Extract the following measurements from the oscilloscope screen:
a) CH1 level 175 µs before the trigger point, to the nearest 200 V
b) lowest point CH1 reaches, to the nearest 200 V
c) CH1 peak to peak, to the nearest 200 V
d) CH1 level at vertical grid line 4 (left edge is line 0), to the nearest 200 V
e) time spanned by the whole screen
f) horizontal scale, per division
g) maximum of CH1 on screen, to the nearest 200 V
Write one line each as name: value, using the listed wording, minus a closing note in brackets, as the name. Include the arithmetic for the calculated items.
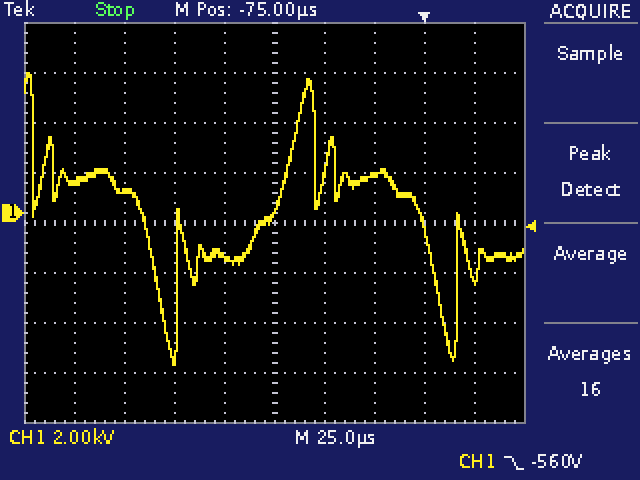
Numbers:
CH1 level 175 µs before the trigger point, to the nearest 200 V: 1.2 kV
lowest point CH1 reaches, to the nearest 200 V: -6.0 kV
CH1 peak to peak, to the nearest 200 V: 5.6 kV − (-6.0 kV) = 11.6 kV
CH1 level at vertical grid line 4 (left edge is line 0), to the nearest 200 V: -1.8 kV
time spanned by the whole screen: 250 µs
horizontal scale, per division: 25 µs
maximum of CH1 on screen, to the nearest 200 V: 5.6 kV
